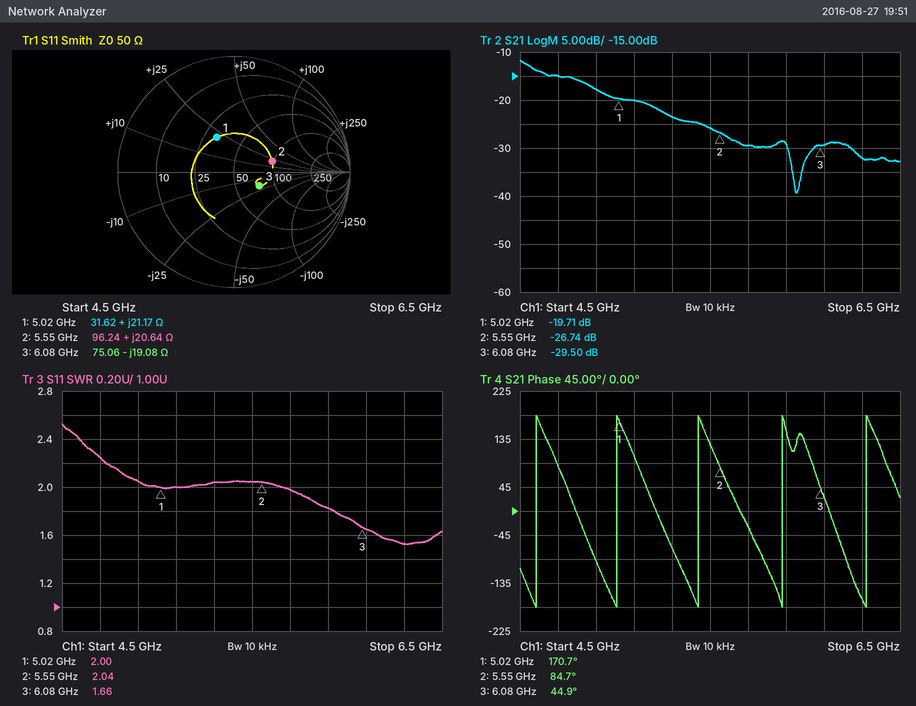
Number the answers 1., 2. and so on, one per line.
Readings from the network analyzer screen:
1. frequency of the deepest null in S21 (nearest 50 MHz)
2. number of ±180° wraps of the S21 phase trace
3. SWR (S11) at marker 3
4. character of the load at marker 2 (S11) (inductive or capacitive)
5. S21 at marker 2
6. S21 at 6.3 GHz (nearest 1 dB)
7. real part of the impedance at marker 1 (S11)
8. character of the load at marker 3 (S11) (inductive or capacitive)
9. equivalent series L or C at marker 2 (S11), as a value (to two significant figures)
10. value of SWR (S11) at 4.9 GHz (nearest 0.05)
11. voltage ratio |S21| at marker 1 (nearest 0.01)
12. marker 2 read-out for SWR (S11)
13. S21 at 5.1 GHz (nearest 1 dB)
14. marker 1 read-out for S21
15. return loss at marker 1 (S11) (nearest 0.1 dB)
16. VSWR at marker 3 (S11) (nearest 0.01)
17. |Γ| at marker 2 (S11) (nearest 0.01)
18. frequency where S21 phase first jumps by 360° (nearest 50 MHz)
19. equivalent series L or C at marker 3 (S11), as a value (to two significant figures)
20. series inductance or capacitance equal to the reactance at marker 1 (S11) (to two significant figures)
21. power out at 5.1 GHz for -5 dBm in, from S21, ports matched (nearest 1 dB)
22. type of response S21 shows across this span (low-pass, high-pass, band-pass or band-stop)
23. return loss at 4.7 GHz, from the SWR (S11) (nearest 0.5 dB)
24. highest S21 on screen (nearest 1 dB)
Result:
1. 5.95 GHz
2. 5
3. 1.66
4. inductive
5. -26.74 dB
6. -32 dB
7. 31.62 Ω
8. capacitive
9. 590 pH
10. 2.05
11. 0.10
12. 2.04
13. -20 dB
14. -19.71 dB
15. 9.6 dB
16. 1.66
17. 0.34
18. 4.60 GHz
19. 1.4 pF
20. 670 pH
21. -25 dBm
22. low-pass
23. 8.5 dB
24. -12 dB
